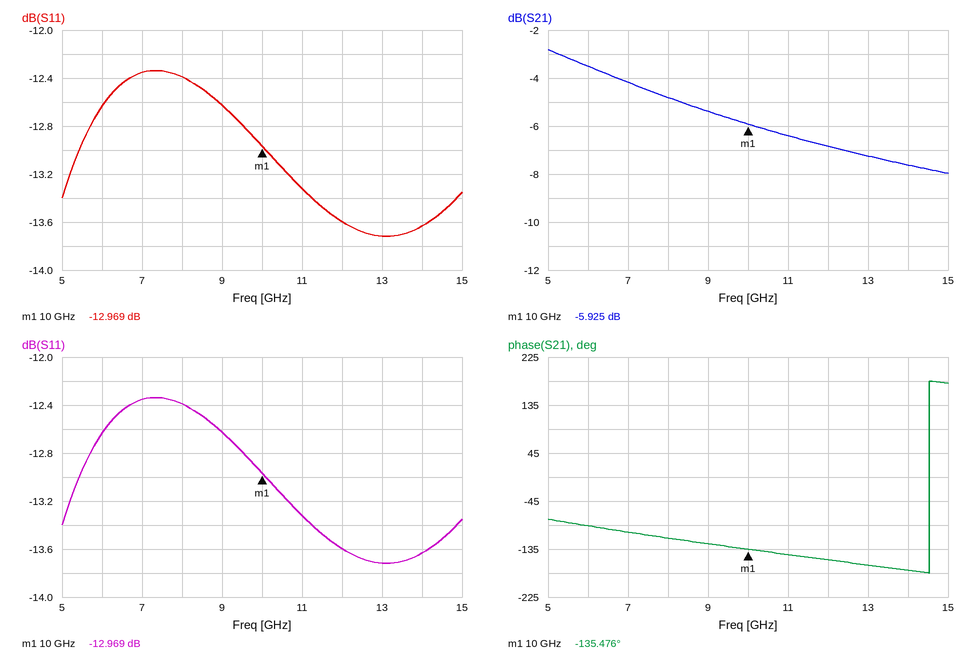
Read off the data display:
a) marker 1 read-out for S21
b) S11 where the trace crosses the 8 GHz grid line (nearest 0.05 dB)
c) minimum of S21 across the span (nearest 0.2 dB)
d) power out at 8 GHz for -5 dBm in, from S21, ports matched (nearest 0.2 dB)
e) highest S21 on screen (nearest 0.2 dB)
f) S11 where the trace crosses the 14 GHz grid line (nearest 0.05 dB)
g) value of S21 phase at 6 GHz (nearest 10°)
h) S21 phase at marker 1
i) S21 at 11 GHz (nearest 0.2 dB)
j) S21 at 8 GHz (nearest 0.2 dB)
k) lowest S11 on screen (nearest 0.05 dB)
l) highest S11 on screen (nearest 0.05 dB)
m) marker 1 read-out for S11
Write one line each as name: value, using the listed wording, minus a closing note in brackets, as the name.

marker 1 read-out for S21: -5.925 dB
S11 where the trace crosses the 8 GHz grid line: -12.40 dB
minimum of S21 across the span: -8.0 dB
power out at 8 GHz for -5 dBm in, from S21, ports matched: -9.8 dBm
highest S21 on screen: -2.8 dB
S11 where the trace crosses the 14 GHz grid line: -13.65 dB
value of S21 phase at 6 GHz: -90°
S21 phase at marker 1: -135.476°
S21 at 11 GHz: -6.4 dB
S21 at 8 GHz: -4.8 dB
lowest S11 on screen: -13.70 dB
highest S11 on screen: -12.35 dB
marker 1 read-out for S11: -12.969 dB
